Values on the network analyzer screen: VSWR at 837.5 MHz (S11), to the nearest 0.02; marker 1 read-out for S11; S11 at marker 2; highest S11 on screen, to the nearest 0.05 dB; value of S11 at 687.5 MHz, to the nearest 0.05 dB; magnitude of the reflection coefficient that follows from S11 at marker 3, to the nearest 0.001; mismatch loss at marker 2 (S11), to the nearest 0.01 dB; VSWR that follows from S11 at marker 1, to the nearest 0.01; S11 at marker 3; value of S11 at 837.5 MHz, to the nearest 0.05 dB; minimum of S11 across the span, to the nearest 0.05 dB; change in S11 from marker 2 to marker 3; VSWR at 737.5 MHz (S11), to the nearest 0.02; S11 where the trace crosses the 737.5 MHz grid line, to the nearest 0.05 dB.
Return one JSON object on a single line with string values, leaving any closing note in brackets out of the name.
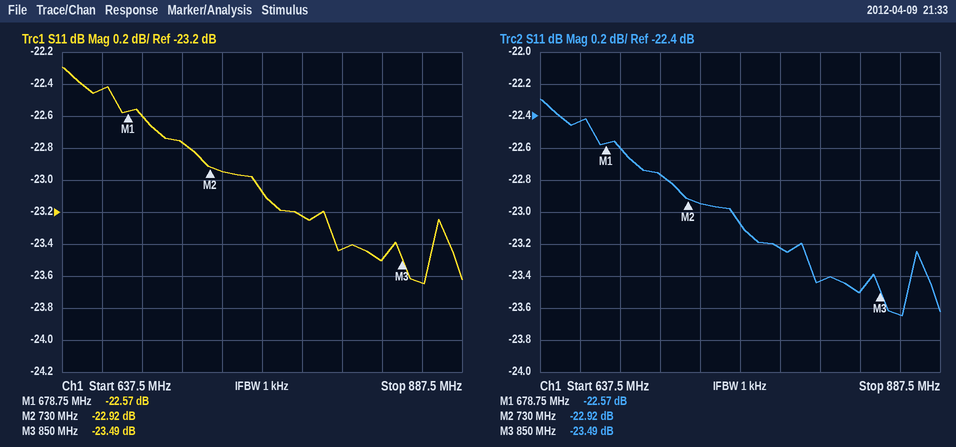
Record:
{"VSWR at 837.5 MHz (S11), to the nearest 0.02": "1.14", "marker 1 read-out for S11": "-22.57 dB", "S11 at marker 2": "-22.92 dB", "highest S11 on screen, to the nearest 0.05 dB": "-22.30 dB", "value of S11 at 687.5 MHz, to the nearest 0.05 dB": "-22.60 dB", "magnitude of the reflection coefficient that follows from S11 at marker 3, to the nearest 0.001": "0.067", "mismatch loss at marker 2 (S11), to the nearest 0.01 dB": "0.02 dB", "VSWR that follows from S11 at marker 1, to the nearest 0.01": "1.16", "S11 at marker 3": "-23.49 dB", "value of S11 at 837.5 MHz, to the nearest 0.05 dB": "-23.50 dB", "minimum of S11 across the span, to the nearest 0.05 dB": "-23.65 dB", "change in S11 from marker 2 to marker 3": "-0.57 dB", "VSWR at 737.5 MHz (S11), to the nearest 0.02": "1.16", "S11 where the trace crosses the 737.5 MHz grid line, to the nearest 0.05 dB": "-22.95 dB"}
